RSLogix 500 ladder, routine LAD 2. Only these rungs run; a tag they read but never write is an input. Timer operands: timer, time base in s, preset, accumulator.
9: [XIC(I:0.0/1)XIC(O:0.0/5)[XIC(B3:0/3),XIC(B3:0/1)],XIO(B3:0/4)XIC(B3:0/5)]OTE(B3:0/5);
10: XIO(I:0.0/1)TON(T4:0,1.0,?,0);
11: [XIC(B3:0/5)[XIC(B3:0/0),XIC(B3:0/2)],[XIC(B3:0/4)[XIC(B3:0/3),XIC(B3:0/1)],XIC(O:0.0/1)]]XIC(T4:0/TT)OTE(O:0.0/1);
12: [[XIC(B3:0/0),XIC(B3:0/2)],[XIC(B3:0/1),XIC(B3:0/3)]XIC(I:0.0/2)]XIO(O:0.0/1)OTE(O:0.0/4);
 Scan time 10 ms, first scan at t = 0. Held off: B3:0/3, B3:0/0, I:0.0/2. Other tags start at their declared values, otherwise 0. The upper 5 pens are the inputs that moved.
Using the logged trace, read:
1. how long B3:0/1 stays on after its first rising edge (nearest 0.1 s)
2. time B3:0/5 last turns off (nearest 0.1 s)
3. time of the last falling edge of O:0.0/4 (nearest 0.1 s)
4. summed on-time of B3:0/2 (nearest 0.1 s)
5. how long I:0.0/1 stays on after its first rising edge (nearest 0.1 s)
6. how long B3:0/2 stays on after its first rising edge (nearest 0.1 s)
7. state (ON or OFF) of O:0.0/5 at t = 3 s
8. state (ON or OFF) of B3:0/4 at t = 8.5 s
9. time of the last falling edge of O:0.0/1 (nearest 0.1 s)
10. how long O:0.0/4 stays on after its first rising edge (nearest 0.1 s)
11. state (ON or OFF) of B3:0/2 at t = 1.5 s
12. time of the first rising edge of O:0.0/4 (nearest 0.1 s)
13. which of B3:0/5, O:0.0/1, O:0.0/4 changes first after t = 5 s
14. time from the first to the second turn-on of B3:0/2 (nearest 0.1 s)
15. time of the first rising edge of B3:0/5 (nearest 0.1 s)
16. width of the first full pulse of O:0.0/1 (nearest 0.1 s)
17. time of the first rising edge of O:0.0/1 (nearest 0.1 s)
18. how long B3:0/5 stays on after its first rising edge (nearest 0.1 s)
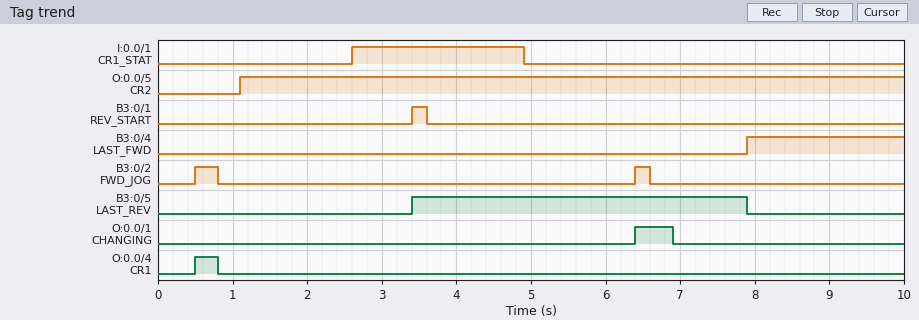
0.2 s
7.9 s
0.8 s
0.5 s
2.3 s
0.3 s
ON
ON
6.9 s
0.3 s
OFF
0.5 s
O:0.0/1
5.9 s
3.4 s
0.5 s
6.4 s
4.5 s
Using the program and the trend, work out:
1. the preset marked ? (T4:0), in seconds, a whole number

2 s
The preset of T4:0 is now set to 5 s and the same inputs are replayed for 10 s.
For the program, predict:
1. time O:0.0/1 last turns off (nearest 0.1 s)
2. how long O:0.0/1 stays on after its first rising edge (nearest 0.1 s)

9.9 s
3.5 s
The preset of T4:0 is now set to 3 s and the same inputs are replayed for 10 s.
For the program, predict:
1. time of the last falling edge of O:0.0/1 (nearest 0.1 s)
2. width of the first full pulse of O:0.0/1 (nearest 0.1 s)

7.9 s
1.5 s
